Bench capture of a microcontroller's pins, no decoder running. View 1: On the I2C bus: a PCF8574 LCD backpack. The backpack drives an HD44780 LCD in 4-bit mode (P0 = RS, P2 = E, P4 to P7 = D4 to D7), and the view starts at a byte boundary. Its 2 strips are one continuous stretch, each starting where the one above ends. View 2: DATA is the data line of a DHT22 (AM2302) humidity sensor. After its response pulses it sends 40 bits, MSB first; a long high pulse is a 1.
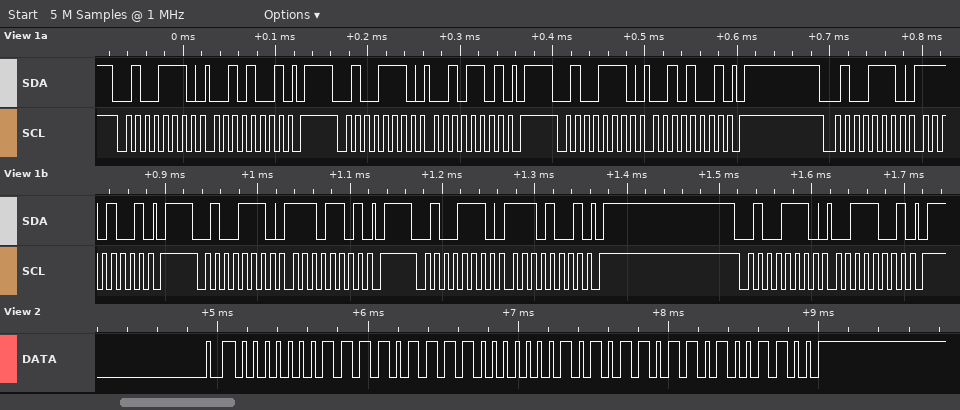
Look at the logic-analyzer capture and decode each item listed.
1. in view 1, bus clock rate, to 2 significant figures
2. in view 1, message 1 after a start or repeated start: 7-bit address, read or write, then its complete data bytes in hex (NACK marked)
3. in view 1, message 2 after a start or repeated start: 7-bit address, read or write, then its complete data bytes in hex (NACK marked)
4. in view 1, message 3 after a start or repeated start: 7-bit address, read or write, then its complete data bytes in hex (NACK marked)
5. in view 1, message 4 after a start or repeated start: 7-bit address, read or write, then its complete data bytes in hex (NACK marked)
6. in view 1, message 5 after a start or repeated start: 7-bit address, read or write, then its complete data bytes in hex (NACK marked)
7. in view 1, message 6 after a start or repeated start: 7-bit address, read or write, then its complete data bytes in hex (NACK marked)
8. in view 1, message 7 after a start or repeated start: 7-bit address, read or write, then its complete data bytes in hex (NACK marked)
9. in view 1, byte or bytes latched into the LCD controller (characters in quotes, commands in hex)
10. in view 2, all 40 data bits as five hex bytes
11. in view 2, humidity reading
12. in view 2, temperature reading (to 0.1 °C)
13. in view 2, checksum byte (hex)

100 kHz
0x27 write: 29
0x27 write: 2D
0x27 write: 29
0x27 write: E9
0x27 write: ED
0x27 write: E9
0x27 write: 39
'.'
01 EF 01 5B 4C
49.5 %
34.7 °C
0x4C
